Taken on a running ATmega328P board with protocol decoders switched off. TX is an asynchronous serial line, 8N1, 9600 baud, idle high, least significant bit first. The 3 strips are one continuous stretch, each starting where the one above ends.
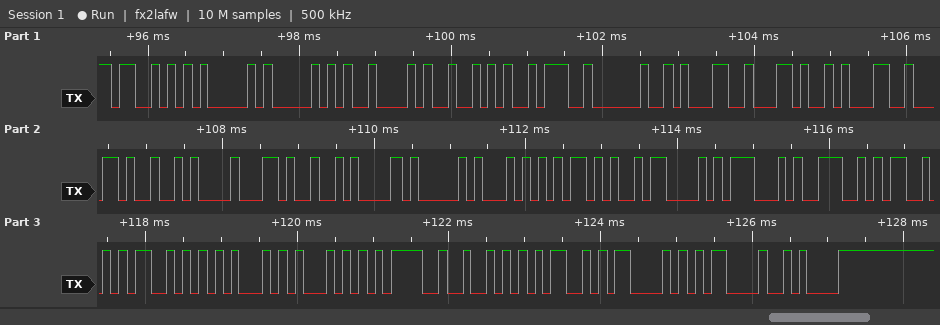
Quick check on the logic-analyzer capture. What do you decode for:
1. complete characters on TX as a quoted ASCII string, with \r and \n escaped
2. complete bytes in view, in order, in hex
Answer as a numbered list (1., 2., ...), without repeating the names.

1. "SAPBR: 1,1,\n,\nAT+CGNSSEQ=RMC\r\n"
2. 53 41 50 42 52 3A 20 31 2C 31 2C 0A 2C 0A 41 54 2B 43 47 4E 53 53 45 51 3D 52 4D 43 0D 0A
